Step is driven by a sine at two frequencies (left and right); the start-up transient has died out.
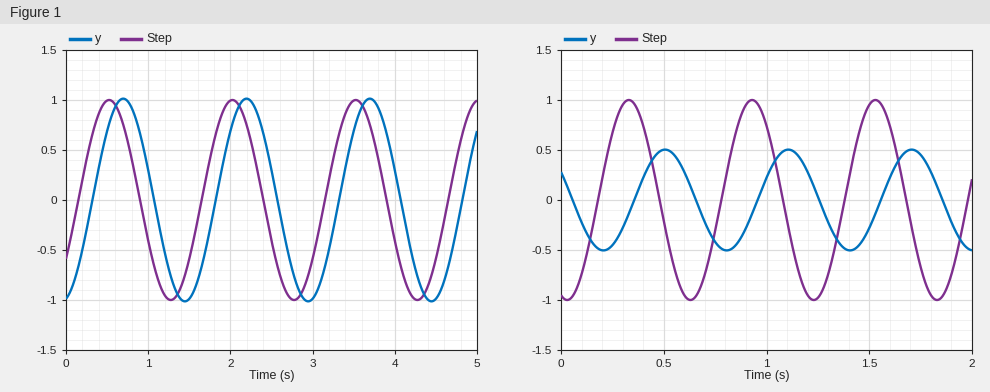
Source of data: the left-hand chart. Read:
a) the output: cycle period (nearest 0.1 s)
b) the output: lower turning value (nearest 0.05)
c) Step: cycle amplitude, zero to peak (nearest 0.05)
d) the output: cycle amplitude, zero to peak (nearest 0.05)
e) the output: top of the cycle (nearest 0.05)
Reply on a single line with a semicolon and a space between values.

1.5 s; -1.00; 1.00; 1.00; 1.00
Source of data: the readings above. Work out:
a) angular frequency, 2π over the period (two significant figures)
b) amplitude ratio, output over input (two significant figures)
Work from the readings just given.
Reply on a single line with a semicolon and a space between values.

4.2 rad/s; 1.0
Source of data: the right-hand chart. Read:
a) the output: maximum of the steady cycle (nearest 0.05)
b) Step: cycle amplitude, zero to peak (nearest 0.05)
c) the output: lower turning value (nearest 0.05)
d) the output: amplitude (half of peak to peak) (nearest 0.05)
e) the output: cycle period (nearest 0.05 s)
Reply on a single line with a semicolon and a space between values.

0.50; 1.00; -0.50; 0.50; 0.60 s
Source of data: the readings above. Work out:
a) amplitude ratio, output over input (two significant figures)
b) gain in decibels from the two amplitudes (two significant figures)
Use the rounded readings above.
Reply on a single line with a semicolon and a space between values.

0.50; -6.0 dB
